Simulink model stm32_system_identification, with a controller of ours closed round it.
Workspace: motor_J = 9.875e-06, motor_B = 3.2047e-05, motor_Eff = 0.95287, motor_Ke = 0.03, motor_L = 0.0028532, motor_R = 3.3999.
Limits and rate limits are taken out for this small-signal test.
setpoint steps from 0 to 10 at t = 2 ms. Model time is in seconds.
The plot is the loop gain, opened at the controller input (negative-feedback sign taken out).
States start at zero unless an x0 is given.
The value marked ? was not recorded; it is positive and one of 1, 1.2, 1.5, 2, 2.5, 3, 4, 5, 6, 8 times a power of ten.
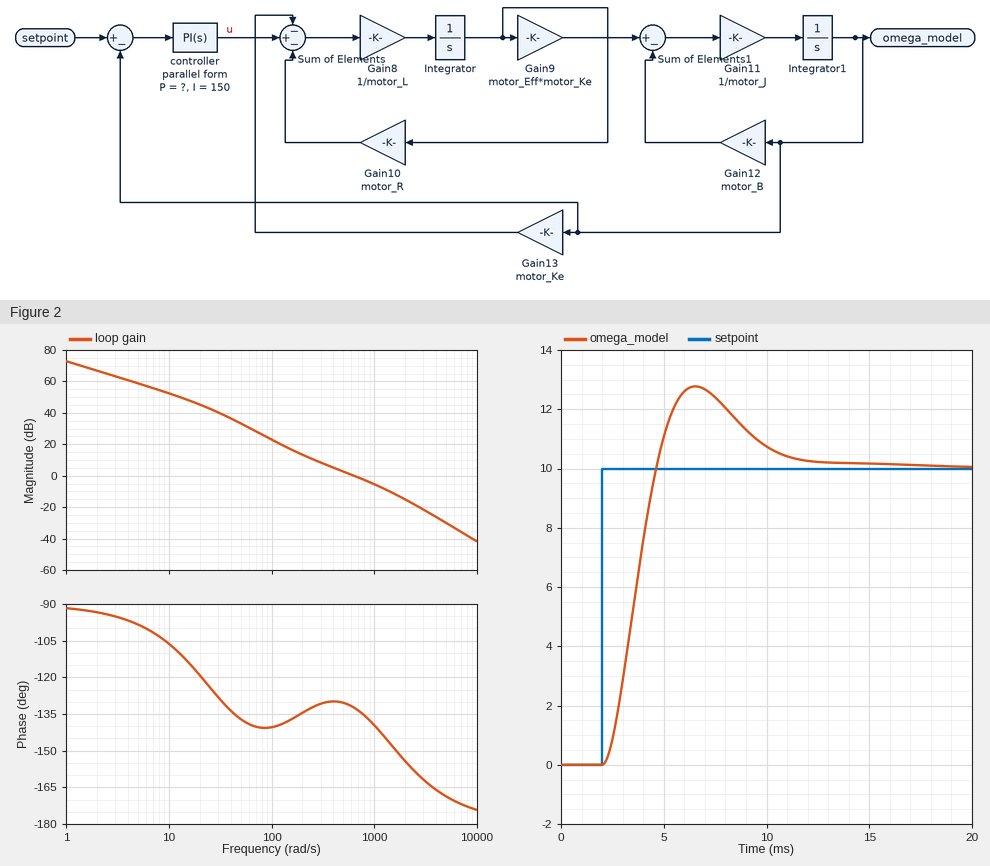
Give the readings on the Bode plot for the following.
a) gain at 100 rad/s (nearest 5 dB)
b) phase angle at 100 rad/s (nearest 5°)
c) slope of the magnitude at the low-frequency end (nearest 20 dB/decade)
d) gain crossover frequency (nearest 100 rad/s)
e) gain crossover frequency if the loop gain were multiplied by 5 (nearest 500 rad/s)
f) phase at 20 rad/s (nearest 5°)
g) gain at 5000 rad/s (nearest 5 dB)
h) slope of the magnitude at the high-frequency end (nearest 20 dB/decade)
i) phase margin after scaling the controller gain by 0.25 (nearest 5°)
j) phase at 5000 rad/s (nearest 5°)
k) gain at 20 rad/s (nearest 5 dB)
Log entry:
25 dB
-140°
-20 dB/decade
600 rad/s
2000 rad/s
-120°
-30 dB
-40 dB/decade
45°
-170°
45 dB
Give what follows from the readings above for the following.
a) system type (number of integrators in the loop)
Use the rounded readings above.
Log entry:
1
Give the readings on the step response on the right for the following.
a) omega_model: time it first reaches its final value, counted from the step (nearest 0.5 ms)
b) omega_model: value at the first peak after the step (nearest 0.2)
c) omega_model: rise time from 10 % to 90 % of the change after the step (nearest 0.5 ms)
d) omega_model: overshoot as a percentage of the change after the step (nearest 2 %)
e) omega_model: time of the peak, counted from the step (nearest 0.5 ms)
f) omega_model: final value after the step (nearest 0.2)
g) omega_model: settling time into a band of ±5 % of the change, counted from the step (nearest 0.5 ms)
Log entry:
2.5 ms
12.8
2.0 ms
28 %
4.5 ms
10.0
8.5 ms
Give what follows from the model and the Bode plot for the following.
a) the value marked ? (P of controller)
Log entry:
0.8
